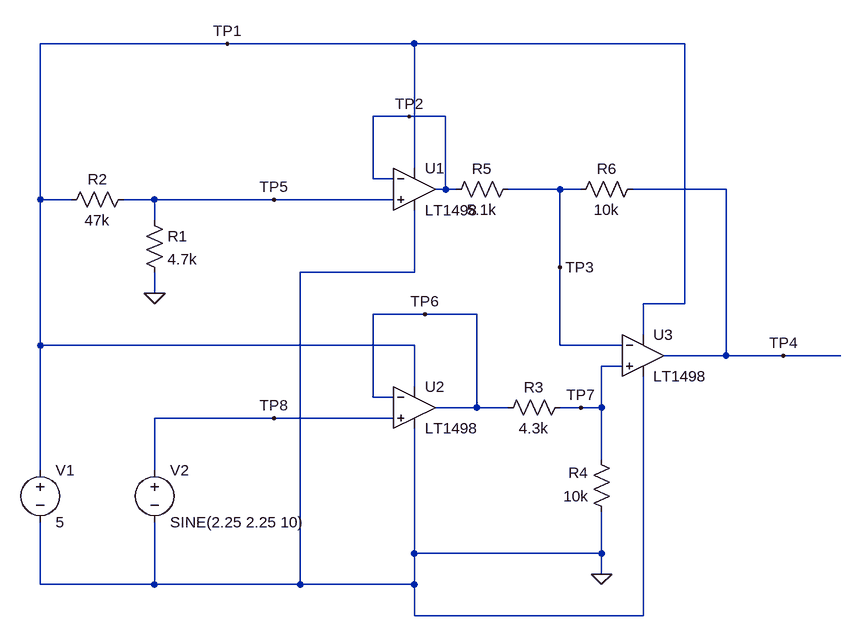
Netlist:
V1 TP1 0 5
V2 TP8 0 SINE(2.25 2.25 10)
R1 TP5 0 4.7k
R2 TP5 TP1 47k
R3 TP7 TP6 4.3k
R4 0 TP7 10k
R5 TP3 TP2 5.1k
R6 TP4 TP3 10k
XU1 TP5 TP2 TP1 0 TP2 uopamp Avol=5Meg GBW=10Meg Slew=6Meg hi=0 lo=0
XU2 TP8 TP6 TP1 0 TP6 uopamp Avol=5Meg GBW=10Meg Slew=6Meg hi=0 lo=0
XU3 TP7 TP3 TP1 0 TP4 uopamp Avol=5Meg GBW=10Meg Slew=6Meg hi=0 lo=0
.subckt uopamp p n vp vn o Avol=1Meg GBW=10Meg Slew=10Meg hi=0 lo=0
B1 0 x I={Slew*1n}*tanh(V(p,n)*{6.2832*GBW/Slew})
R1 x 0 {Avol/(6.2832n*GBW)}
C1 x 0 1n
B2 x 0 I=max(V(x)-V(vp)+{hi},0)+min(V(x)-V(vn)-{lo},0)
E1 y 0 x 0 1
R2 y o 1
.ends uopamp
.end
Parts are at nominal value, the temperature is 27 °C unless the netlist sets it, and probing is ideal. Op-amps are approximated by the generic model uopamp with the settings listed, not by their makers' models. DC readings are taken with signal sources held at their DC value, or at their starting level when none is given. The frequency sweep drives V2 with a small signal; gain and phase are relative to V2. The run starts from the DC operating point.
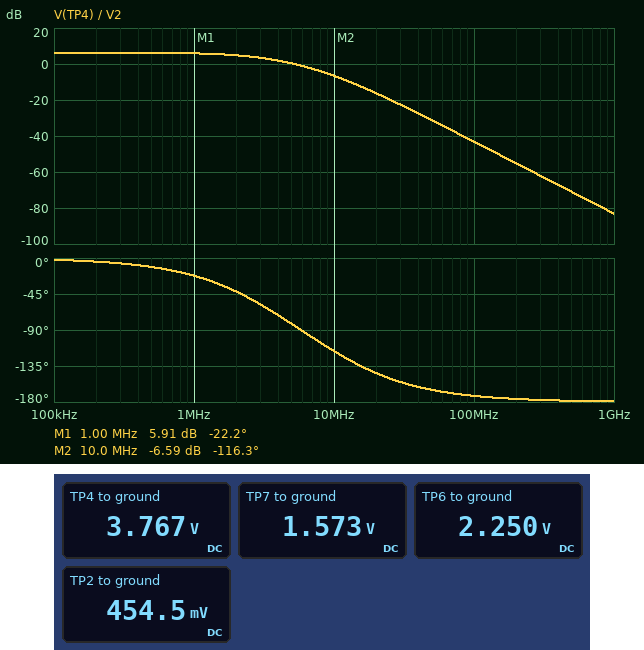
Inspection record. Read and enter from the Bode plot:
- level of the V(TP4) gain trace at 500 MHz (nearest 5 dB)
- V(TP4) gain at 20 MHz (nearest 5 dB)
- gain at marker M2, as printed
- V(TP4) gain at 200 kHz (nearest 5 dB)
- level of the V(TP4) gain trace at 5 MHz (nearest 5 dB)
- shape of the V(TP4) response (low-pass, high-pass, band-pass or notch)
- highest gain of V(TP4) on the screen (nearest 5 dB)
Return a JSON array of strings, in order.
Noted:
["-70 dB", "-15 dB", "-6.59 dB", "5 dB", "0 dB", "low-pass", "5 dB"]
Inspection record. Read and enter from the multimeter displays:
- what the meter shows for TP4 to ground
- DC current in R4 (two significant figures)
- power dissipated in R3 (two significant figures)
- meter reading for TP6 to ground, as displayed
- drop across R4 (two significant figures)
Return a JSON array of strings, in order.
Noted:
["3.767 V", "160 µA", "110 µW", "2.250 V", "1.6 V"]
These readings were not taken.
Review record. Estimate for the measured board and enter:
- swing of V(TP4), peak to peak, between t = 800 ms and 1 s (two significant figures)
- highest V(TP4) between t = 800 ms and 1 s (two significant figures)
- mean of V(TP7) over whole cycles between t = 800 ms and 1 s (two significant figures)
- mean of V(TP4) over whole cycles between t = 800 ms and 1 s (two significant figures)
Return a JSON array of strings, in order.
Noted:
["5.0 V", "5.0 V", "1.6 V", "3.0 V"]
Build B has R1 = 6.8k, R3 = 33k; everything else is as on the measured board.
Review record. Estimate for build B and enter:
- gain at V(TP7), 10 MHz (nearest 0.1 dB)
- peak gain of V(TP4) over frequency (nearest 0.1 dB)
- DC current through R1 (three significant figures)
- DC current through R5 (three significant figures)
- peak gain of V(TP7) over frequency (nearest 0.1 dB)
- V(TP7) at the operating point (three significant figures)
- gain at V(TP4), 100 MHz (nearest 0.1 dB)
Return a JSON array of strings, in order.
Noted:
["-15.7 dB", "-3.2 dB", "92.9 µA", "21.3 µA", "-12.7 dB", "523 mV", "-52.7 dB"]
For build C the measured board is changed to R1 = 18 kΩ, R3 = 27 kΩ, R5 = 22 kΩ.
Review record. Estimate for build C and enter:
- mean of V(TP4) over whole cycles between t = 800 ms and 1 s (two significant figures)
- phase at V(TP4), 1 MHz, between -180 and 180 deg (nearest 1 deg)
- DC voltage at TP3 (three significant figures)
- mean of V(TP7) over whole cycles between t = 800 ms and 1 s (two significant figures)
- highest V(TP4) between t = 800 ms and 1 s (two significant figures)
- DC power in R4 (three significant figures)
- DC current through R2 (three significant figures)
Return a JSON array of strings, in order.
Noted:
["420 mV", "-14 deg", "608 mV", "610 mV", "1.1 V", "37.0 µW", "76.9 µA"]
